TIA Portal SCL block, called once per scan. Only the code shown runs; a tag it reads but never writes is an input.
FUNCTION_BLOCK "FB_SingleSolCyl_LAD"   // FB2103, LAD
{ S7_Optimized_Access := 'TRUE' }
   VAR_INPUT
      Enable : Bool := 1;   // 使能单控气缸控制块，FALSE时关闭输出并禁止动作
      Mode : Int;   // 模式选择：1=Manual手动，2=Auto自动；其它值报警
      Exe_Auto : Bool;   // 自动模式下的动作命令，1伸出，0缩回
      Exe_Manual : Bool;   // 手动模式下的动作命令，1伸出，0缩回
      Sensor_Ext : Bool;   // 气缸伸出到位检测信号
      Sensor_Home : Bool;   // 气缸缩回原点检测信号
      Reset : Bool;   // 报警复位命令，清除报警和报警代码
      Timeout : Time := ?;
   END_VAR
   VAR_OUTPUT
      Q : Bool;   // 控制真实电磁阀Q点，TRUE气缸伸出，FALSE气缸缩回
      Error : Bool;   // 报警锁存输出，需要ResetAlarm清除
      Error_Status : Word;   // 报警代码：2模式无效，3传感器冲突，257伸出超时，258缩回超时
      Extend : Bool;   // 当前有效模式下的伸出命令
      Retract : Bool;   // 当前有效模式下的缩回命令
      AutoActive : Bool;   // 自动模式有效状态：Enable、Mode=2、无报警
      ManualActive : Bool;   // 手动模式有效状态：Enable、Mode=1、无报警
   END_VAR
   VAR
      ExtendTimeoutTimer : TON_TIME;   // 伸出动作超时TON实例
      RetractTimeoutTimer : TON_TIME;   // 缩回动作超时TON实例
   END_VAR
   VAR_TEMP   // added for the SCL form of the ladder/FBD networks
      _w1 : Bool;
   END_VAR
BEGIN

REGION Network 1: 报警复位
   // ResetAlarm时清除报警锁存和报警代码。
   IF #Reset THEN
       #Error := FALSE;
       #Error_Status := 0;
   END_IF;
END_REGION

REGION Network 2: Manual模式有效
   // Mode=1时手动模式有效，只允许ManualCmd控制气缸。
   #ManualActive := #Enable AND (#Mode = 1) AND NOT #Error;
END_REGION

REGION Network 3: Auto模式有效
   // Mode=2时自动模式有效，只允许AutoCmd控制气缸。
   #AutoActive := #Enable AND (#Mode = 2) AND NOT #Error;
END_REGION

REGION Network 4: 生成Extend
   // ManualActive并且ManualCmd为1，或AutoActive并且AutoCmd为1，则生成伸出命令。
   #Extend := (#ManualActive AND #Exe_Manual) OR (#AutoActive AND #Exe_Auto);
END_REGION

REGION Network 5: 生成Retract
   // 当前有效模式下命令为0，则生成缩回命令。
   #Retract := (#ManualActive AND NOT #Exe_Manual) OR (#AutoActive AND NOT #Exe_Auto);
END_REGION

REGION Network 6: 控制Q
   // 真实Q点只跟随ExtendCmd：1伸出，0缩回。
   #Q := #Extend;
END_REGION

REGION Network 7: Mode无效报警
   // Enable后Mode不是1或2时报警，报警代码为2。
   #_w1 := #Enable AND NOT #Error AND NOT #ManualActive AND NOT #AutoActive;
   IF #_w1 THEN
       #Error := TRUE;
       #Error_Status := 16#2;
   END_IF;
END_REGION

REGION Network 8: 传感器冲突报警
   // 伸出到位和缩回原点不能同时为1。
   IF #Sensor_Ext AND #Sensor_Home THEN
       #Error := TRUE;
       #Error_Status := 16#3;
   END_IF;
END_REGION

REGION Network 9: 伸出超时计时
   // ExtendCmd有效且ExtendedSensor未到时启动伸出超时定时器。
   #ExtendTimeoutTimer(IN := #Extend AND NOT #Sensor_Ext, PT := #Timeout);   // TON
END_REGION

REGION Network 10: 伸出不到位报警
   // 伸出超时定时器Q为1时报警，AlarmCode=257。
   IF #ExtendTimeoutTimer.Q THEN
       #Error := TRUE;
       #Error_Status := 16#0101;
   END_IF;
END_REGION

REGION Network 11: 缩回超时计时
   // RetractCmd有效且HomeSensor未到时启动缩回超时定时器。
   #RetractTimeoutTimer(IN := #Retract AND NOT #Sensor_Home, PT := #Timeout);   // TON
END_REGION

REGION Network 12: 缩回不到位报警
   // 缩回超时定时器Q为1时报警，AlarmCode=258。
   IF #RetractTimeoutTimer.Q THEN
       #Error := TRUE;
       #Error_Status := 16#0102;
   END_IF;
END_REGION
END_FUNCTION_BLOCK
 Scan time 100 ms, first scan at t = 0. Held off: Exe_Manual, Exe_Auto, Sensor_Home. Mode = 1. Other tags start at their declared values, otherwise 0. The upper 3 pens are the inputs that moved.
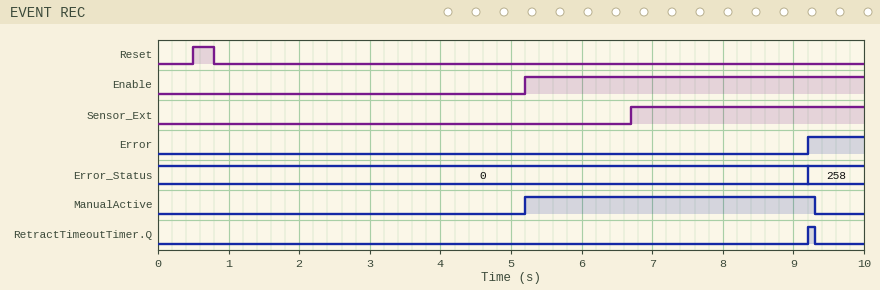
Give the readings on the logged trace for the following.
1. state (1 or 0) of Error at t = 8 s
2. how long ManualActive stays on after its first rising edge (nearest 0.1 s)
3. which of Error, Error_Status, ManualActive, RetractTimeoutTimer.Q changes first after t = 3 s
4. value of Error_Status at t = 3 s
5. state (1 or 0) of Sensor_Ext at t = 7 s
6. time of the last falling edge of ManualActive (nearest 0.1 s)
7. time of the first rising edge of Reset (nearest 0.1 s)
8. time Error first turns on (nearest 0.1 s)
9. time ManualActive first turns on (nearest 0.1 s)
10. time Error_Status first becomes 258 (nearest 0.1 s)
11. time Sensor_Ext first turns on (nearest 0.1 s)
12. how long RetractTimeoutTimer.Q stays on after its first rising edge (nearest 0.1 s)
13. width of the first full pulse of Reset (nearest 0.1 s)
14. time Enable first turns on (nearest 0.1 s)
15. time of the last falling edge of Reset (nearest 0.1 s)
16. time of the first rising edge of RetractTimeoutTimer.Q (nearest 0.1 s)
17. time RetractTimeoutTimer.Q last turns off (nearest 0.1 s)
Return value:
0
4.1 s
ManualActive
0
1
9.3 s
0.5 s
9.2 s
5.2 s
9.2 s
6.7 s
0.1 s
0.3 s
5.2 s
0.8 s
9.2 s
9.3 s
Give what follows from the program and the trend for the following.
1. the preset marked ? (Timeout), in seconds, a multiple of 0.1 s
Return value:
4.0 s
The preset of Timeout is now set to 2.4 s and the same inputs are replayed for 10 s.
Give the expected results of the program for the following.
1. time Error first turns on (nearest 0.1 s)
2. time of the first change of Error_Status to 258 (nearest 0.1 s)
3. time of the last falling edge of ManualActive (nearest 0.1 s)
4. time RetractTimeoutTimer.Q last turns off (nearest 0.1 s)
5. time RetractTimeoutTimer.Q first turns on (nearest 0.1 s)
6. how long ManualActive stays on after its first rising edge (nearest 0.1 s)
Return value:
7.6 s
7.6 s
7.7 s
7.7 s
7.6 s
2.5 s
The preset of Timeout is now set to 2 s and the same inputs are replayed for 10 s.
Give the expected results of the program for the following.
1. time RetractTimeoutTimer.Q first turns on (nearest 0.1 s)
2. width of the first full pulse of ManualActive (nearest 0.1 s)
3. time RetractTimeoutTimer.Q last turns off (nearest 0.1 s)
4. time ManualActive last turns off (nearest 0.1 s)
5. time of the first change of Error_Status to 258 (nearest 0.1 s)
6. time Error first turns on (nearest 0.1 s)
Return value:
7.2 s
2.1 s
7.3 s
7.3 s
7.2 s
7.2 s
